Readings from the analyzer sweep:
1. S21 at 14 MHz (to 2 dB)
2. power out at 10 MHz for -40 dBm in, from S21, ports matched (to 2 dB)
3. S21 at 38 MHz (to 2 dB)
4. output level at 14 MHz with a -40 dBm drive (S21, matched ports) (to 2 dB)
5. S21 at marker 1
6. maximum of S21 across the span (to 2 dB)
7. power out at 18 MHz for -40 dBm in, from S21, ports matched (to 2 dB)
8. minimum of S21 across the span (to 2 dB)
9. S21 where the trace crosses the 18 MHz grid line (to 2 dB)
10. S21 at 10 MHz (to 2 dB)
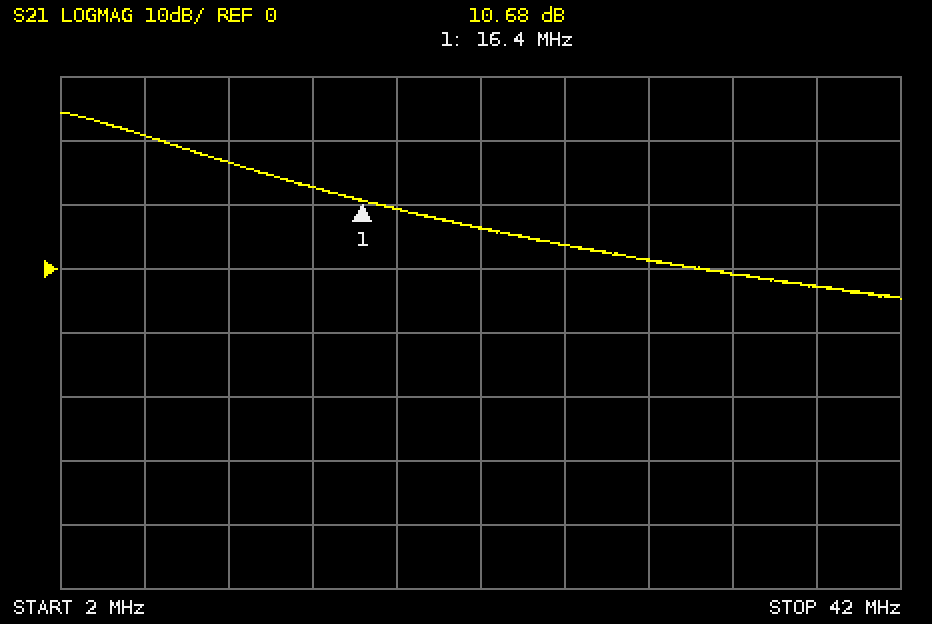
12 dB
-24 dBm
-2 dB
-28 dBm
10.68 dB
24 dB
-30 dBm
-4 dB
10 dB
16 dB
